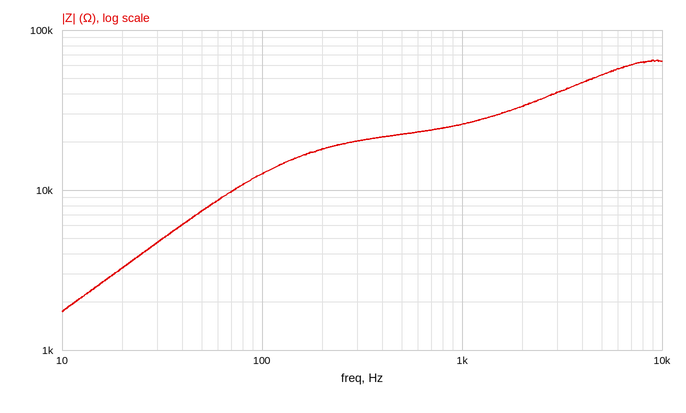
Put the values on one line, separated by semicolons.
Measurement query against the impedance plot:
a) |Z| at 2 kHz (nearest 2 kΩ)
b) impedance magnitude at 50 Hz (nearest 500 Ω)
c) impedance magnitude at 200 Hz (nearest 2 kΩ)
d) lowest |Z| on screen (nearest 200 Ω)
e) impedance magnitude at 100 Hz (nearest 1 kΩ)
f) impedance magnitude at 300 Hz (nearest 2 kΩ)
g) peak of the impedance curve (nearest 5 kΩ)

34 kΩ; 7.5 kΩ; 18 kΩ; 1.8 kΩ; 13 kΩ; 20 kΩ; 65 kΩ
